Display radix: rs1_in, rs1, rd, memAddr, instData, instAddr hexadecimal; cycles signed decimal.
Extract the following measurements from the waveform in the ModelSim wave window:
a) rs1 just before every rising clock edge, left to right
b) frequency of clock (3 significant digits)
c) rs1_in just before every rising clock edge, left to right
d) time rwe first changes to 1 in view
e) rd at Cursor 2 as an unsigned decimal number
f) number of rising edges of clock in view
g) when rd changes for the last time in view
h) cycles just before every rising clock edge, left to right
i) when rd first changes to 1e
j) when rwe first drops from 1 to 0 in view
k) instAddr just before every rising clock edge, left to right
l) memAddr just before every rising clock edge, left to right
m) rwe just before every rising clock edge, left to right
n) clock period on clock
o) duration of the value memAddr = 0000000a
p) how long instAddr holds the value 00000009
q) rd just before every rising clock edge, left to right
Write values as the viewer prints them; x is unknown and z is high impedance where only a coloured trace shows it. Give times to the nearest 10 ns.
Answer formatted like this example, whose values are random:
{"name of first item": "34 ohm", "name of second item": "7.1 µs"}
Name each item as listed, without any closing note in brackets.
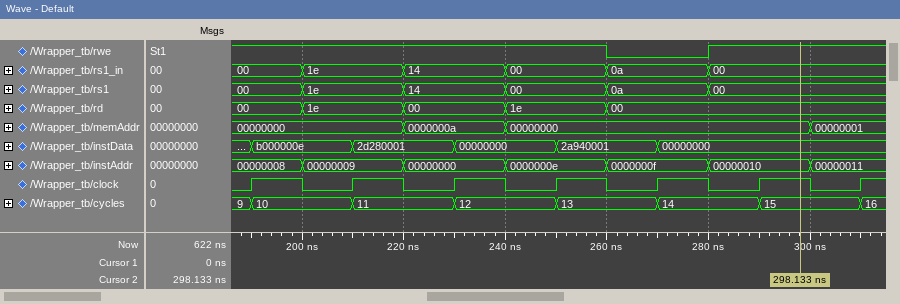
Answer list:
{"rs1 just before every rising clock edge, left to right": "00, 1e, 14, 00, 0a, 00, 00", "frequency of clock": "50.0 MHz", "rs1_in just before every rising clock edge, left to right": "00, 1e, 14, 00, 0a, 00, 00", "time rwe first changes to 1 in view": "280 ns", "rd at Cursor 2 as an unsigned decimal number": "0", "number of rising edges of clock in view": "7", "when rd changes for the last time in view": "260 ns", "cycles just before every rising clock edge, left to right": "9, 10, 11, 12, 13, 14, 15", "when rd first changes to 1e": "200 ns", "when rwe first drops from 1 to 0 in view": "260 ns", "instAddr just before every rising clock edge, left to right": "00000008, 00000009, 00000000, 0000000e, 0000000f, 00000010, 00000011", "memAddr just before every rising clock edge, left to right": "00000000, 00000000, 0000000a, 00000000, 00000000, 00000000, 00000001", "rwe just before every rising clock edge, left to right": "1 1 1 1 0 1 1", "clock period on clock": "20 ns", "duration of the value memAddr = 0000000a": "20 ns", "how long instAddr holds the value 00000009": "20 ns", "rd just before every rising clock edge, left to right": "00, 1e, 00, 1e, 00, 00, 00"}
